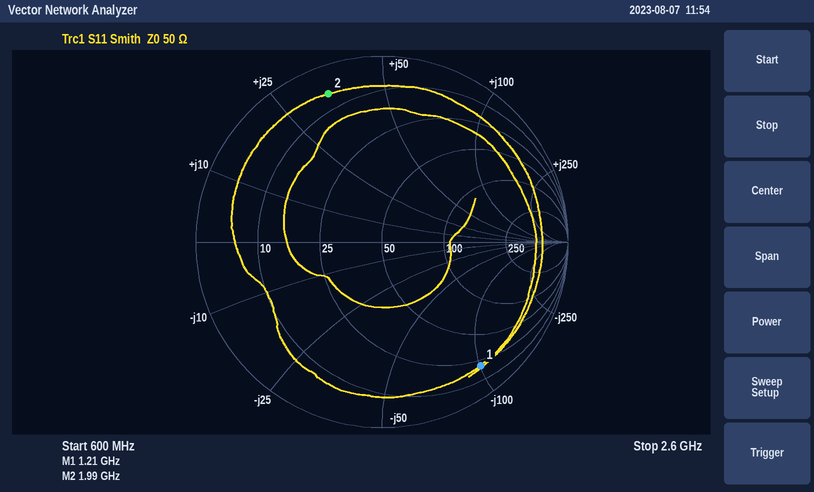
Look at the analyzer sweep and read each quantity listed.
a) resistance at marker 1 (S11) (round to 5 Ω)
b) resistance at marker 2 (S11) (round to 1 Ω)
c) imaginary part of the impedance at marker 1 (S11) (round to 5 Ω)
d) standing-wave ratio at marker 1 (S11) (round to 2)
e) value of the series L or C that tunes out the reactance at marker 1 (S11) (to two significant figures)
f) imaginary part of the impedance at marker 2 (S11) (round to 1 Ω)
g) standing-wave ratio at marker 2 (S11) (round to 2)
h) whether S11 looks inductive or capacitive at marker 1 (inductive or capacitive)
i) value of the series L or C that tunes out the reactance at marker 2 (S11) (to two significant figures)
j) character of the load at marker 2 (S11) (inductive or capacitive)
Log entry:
20 Ω
6 Ω
-100 Ω
12
13 nH
+35 Ω
12
capacitive
2.3 pF
inductive
